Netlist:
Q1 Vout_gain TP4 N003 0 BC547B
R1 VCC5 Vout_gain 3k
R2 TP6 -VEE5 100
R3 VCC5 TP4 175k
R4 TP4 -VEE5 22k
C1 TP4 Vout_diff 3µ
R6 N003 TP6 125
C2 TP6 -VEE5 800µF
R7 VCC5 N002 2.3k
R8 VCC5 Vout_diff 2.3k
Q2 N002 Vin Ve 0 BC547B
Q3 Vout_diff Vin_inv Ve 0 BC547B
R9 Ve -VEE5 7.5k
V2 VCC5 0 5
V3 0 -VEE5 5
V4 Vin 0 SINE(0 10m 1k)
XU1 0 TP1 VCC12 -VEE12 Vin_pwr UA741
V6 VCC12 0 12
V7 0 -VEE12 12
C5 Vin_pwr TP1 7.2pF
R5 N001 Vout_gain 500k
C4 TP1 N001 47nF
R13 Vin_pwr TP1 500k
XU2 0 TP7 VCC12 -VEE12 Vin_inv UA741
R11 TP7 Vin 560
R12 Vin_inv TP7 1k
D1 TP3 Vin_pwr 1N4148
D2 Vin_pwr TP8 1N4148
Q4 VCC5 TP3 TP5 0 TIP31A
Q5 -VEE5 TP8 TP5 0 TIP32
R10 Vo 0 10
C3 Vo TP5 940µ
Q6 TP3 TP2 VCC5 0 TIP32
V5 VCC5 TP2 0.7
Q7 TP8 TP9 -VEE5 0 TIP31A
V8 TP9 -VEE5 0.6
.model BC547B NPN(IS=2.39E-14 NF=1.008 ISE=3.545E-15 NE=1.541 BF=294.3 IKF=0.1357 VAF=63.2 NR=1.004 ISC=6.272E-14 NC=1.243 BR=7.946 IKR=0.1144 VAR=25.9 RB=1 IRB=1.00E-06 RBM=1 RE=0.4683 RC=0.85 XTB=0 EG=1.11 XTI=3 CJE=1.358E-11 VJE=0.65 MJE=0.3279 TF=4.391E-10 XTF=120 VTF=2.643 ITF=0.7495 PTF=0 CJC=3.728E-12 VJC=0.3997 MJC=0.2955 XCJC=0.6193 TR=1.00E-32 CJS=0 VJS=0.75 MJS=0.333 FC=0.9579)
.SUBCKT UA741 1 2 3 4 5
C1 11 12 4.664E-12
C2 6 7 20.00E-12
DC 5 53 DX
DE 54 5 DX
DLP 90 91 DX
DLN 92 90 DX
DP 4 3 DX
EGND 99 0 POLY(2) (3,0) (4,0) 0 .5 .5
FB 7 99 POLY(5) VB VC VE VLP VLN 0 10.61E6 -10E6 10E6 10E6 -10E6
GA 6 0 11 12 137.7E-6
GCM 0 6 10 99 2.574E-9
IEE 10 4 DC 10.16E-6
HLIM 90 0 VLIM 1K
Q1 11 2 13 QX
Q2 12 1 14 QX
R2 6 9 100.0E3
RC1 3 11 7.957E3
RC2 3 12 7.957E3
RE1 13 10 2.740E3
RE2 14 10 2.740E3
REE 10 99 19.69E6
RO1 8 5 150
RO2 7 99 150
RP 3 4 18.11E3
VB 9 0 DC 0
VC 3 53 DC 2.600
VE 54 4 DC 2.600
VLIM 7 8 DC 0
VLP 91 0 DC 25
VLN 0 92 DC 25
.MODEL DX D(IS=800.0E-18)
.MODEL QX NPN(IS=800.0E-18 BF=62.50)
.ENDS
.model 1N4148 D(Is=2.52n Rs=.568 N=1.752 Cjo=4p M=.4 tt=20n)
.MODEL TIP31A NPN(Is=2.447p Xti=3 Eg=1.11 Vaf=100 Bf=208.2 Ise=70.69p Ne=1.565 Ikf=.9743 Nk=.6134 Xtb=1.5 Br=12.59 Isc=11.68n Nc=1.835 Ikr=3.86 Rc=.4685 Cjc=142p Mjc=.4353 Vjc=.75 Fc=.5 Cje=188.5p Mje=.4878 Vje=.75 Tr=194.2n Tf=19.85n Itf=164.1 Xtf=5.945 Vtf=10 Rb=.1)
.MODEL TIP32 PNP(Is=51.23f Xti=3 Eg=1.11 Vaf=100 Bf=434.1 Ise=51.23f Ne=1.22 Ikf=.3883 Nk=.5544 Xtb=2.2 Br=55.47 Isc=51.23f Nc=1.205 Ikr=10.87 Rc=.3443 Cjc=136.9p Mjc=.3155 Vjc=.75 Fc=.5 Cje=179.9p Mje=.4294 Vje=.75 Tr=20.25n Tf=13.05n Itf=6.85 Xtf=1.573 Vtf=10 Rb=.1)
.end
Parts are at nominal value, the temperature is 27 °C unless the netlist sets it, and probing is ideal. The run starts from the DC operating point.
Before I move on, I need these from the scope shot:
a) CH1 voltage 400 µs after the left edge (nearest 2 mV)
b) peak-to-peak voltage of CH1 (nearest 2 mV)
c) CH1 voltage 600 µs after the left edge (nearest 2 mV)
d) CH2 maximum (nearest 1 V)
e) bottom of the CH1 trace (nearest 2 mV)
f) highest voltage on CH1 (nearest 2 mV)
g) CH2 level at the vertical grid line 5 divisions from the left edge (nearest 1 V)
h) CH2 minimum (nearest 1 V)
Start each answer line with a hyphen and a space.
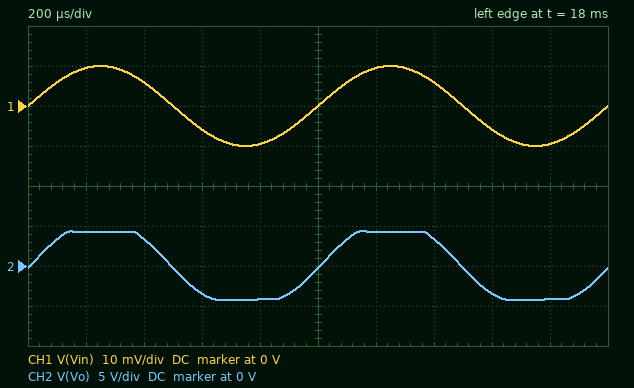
- 6 mV
- 20 mV
- -6 mV
- 4 V
- -10 mV
- 10 mV
- 0 V
- -4 V
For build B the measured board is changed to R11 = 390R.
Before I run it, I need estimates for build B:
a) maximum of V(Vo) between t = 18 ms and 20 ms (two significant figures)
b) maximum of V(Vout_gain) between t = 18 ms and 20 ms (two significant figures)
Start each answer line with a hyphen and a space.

- 4.4 V
- 5.0 V
